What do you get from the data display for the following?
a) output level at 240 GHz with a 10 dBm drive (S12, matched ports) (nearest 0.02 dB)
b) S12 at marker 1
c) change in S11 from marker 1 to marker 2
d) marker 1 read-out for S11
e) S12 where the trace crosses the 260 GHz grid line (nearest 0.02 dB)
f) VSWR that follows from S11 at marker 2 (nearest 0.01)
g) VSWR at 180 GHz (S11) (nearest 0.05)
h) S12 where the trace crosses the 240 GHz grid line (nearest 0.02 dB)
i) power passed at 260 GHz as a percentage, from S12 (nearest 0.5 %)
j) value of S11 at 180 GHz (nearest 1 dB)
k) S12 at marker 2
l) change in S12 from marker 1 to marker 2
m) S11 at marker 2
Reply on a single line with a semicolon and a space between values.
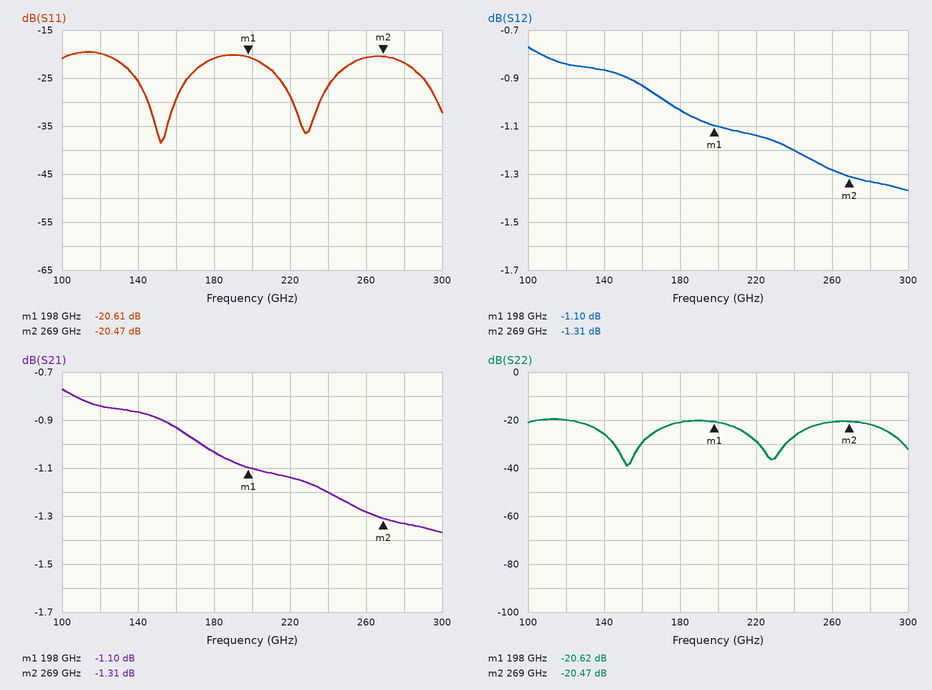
8.80 dBm; -1.10 dB; 0.14 dB; -20.61 dB; -1.28 dB; 1.21; 1.20; -1.20 dB; 74.5 %; -21 dB; -1.31 dB; -0.21 dB; -20.47 dB
